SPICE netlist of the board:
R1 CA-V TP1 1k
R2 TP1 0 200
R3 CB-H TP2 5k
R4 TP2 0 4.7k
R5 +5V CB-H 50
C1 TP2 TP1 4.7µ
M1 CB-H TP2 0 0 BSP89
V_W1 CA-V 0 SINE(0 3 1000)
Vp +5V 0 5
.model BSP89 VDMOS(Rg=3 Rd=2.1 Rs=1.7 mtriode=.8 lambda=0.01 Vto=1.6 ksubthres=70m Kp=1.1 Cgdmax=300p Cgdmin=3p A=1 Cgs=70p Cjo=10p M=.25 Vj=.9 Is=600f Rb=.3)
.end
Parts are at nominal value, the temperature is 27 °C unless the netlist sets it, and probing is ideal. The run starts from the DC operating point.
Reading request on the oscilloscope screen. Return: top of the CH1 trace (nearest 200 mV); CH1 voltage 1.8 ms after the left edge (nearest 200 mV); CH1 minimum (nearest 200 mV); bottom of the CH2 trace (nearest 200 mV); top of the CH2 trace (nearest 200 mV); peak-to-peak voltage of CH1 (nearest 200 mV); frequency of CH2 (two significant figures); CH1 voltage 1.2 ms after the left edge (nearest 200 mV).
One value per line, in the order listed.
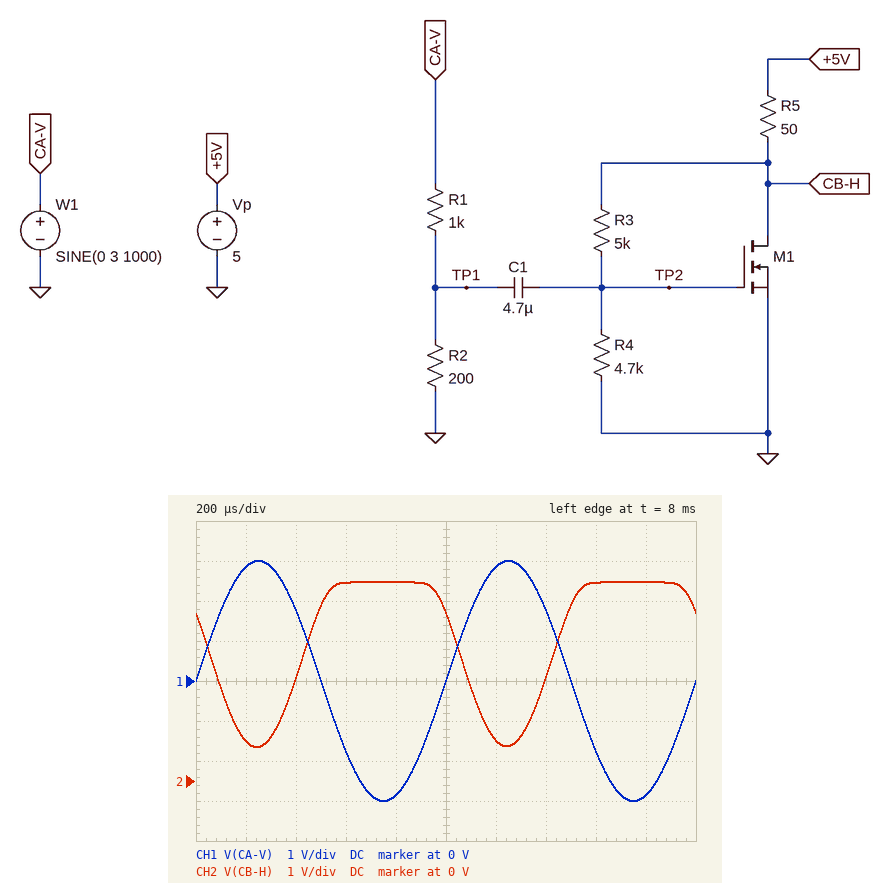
3.0 V
-2.8 V
-3.0 V
800 mV
5.0 V
6.0 V
1.0 kHz
2.8 V
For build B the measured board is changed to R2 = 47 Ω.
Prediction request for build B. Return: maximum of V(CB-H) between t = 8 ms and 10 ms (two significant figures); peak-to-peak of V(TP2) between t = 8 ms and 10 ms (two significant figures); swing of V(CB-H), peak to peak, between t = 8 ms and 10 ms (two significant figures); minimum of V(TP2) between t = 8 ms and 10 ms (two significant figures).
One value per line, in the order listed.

4.6 V
250 mV
1.8 V
1.7 V
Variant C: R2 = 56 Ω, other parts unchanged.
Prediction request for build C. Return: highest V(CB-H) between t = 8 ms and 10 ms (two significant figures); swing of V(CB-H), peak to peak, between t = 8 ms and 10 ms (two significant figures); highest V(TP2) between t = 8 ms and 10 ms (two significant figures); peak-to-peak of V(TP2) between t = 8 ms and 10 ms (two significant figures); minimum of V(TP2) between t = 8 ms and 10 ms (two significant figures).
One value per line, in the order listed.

4.7 V
2.1 V
2.0 V
290 mV
1.7 V
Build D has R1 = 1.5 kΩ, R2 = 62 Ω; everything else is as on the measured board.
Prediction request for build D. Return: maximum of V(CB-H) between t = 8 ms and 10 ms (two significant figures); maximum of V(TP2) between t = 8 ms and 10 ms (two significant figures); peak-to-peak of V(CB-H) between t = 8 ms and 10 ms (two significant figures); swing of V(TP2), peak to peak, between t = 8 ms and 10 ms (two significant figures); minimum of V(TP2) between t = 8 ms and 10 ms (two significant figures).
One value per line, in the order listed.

4.5 V
1.9 V
1.6 V
210 mV
1.7 V
